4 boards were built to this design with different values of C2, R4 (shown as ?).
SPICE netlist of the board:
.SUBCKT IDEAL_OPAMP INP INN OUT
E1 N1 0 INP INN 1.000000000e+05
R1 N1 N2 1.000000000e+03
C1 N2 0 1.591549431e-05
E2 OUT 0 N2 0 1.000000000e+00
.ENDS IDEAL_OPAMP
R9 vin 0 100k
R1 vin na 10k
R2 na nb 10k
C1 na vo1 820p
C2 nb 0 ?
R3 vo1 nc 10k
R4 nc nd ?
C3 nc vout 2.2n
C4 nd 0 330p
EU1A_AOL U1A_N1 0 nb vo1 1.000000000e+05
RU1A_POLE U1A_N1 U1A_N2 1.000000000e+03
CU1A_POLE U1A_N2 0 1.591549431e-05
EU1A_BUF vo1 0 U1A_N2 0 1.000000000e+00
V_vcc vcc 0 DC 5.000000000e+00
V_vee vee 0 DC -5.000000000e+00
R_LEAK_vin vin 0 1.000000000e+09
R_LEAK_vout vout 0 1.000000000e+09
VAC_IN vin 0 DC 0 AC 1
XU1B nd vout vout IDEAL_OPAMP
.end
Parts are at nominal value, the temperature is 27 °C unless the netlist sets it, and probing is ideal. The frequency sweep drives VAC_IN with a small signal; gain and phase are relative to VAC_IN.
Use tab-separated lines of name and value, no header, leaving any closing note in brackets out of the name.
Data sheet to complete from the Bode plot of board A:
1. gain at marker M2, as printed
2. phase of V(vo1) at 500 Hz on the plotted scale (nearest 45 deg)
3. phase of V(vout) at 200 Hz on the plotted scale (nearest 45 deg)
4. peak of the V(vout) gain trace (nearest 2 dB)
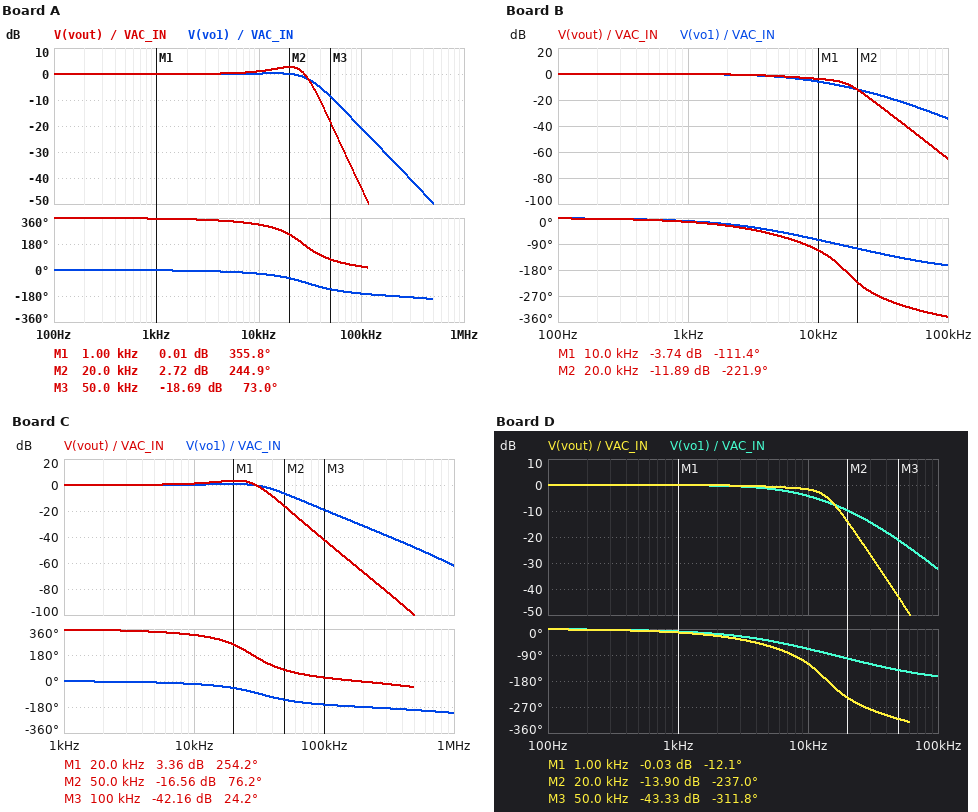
gain at marker M2, as printed	2.72 dB
phase of V(vo1) at 500 Hz on the plotted scale	0 deg
phase of V(vout) at 200 Hz on the plotted scale	360 deg
peak of the V(vout) gain trace	2 dB
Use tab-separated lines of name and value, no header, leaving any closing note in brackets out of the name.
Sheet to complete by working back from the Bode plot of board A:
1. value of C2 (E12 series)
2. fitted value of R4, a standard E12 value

value of C2	330 pF
fitted value of R4, a standard E12 value	4.7 kΩ
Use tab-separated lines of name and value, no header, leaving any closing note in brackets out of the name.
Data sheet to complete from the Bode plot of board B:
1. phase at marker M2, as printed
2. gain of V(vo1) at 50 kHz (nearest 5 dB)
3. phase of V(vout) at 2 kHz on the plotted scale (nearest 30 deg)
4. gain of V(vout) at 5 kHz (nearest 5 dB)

phase at marker M2, as printed	-221.9 deg
gain of V(vo1) at 50 kHz	-25 dB
phase of V(vout) at 2 kHz on the plotted scale	-30 deg
gain of V(vout) at 5 kHz	0 dB
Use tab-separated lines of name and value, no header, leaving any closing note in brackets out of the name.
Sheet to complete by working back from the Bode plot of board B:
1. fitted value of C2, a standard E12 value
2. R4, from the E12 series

fitted value of C2, a standard E12 value	1.5 nF
R4, from the E12 series	12 kΩ
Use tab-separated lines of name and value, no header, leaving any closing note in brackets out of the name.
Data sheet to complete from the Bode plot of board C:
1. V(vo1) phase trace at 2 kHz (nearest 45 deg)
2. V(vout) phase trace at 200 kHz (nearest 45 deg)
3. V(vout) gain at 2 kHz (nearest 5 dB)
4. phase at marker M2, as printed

V(vo1) phase trace at 2 kHz	0 deg
V(vout) phase trace at 200 kHz	0 deg
V(vout) gain at 2 kHz	0 dB
phase at marker M2, as printed	76.2 deg
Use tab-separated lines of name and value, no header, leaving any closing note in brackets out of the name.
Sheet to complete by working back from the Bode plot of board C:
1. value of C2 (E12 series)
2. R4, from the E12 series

value of C2	270 pF
R4, from the E12 series	4.7 kΩ
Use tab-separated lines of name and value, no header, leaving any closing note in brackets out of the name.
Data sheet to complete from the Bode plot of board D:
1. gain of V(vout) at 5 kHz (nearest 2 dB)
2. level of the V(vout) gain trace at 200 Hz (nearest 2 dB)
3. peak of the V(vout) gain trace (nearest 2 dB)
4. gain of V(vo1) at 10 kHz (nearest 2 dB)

gain of V(vout) at 5 kHz	0 dB
level of the V(vout) gain trace at 200 Hz	0 dB
peak of the V(vout) gain trace	0 dB
gain of V(vo1) at 10 kHz	-4 dB
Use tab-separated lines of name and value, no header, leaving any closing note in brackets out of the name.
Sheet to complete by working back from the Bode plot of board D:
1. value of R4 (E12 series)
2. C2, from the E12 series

value of R4	18 kΩ
C2, from the E12 series	1.2 nF
